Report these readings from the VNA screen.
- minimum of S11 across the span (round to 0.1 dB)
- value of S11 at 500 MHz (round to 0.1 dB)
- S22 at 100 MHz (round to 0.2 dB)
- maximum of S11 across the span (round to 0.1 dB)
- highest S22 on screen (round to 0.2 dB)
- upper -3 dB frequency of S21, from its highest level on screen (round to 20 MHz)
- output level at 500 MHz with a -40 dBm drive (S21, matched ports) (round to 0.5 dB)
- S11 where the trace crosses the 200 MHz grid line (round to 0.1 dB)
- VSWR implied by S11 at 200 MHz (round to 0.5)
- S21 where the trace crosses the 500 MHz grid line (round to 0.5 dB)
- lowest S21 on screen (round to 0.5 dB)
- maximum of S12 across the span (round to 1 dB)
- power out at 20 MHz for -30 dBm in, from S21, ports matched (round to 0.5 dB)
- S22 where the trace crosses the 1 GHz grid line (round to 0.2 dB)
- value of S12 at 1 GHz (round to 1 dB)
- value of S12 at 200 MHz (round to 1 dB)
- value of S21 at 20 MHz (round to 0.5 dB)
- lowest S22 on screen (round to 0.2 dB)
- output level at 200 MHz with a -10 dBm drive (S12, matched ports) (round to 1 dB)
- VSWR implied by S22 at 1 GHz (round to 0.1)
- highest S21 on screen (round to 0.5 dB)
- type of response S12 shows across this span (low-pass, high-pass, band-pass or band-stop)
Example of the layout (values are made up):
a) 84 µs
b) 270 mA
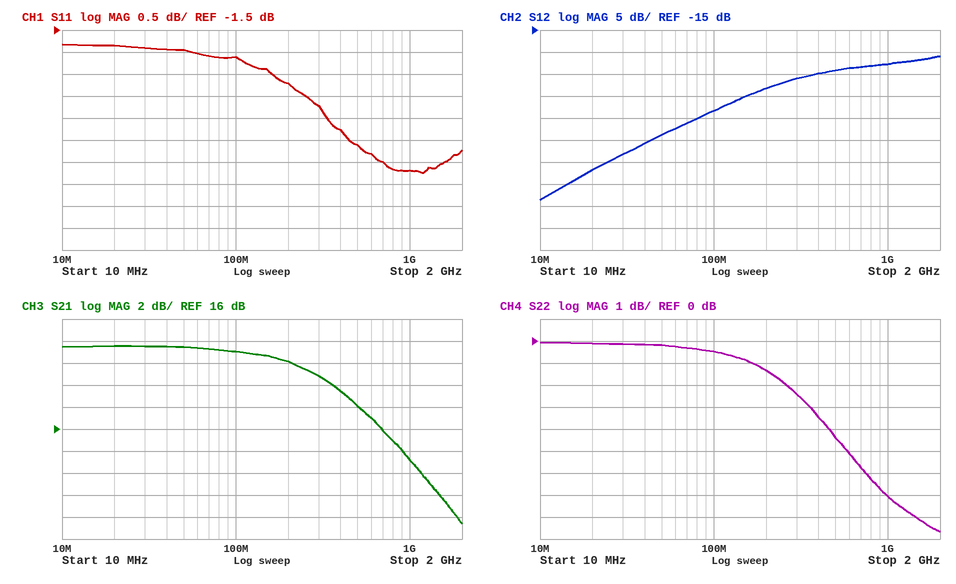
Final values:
a) -4.7 dB
b) -4.1 dB
c) -0.4 dB
d) -1.8 dB
e) 0.0 dB
f) 320 MHz
g) -22.0 dBm
h) -2.7 dB
i) 6.5
j) 18.0 dB
k) 7.5 dB
l) -21 dB
m) -6.5 dBm
n) -7.0 dB
o) -23 dB
p) -28 dB
q) 23.5 dB
r) -8.6 dB
s) -38 dBm
t) 2.6
u) 23.5 dB
v) high-pass
